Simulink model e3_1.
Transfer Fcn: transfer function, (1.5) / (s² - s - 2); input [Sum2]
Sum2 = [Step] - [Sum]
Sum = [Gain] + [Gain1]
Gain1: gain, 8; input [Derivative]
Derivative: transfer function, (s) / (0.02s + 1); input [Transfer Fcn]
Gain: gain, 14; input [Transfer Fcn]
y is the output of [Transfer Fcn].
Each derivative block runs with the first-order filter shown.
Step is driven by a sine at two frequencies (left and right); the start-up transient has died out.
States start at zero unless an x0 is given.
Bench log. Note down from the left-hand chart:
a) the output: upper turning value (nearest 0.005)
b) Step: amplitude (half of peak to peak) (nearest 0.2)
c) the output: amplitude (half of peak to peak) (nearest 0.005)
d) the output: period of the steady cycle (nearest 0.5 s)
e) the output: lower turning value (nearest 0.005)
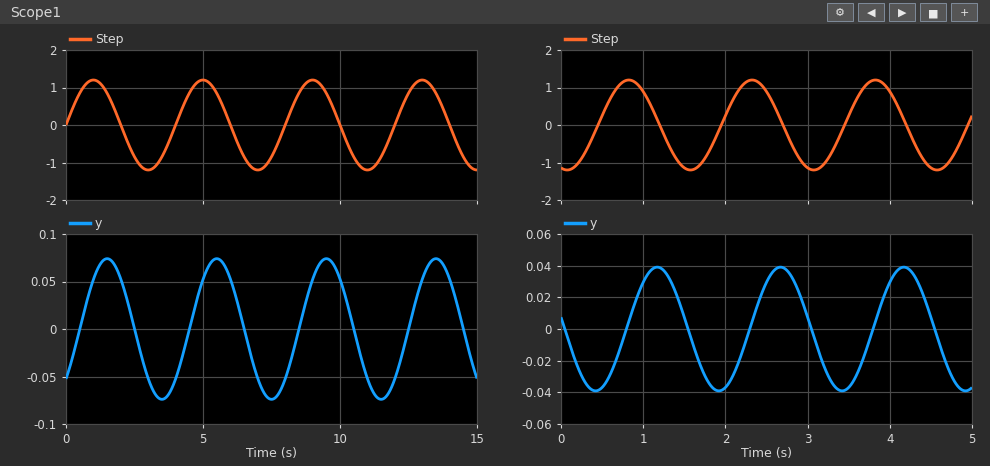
0.075
1.2
0.075
4.0 s
-0.075
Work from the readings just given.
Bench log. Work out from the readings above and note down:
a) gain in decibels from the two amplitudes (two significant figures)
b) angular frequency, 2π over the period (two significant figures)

-24 dB
1.6 rad/s
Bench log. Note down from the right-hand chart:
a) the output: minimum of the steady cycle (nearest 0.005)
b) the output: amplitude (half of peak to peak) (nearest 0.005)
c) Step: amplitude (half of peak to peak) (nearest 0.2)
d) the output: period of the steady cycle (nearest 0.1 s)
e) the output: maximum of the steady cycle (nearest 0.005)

-0.040
0.040
1.2
1.5 s
0.040
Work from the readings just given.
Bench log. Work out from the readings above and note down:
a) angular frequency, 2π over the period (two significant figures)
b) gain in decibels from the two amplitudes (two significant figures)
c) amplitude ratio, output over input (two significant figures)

4.2 rad/s
-30 dB
0.033
